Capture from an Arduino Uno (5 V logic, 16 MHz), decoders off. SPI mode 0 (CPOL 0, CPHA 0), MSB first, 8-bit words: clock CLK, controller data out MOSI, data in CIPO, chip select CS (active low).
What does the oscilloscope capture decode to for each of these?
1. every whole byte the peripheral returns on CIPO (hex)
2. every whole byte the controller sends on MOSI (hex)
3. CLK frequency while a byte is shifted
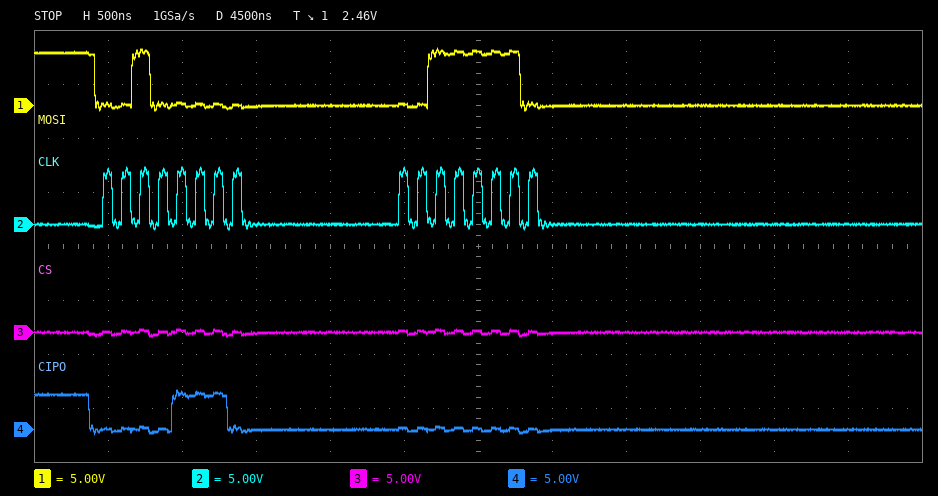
0E 00
20 3E
8 MHz
